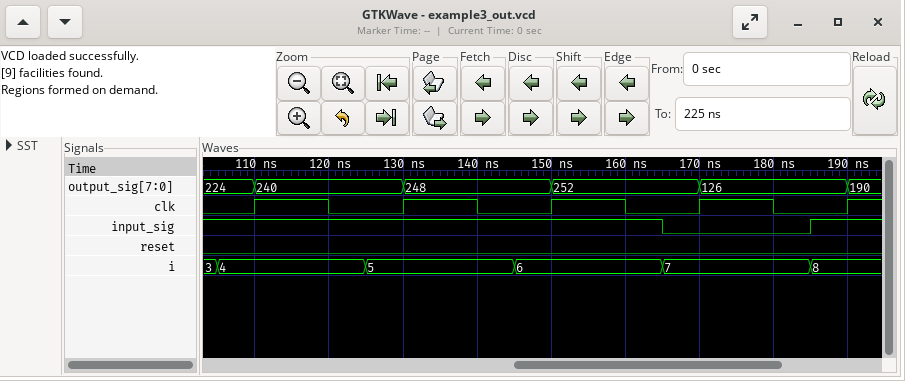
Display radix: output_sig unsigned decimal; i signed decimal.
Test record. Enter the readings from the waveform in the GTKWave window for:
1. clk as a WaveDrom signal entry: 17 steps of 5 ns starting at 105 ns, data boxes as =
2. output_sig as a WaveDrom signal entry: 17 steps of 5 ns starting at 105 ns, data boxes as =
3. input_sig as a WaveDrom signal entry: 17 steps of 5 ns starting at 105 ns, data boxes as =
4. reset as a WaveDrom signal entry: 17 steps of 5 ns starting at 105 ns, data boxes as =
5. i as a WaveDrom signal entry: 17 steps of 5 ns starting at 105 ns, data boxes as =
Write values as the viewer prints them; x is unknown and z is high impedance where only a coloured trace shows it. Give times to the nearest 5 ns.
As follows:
{name: 'clk', wave: '01.0.1.0.1.0.1.0.'}
{name: 'output_sig', wave: '==...=...=...=...', data: '224 240 248 252 126'}
{name: 'input_sig', wave: '1...........0...1'}
{name: 'reset', wave: '0................'}
{name: 'i', wave: '=...=...=...=...=', data: '4 5 6 7 8'}
